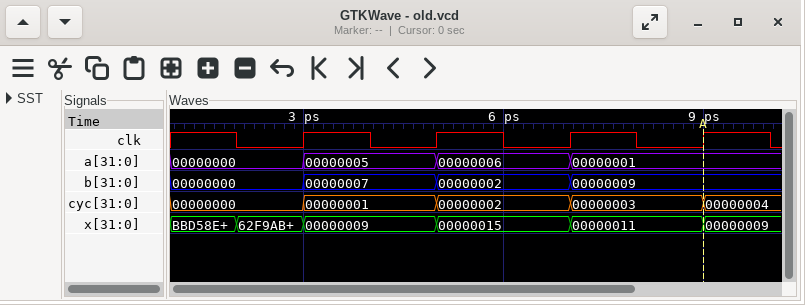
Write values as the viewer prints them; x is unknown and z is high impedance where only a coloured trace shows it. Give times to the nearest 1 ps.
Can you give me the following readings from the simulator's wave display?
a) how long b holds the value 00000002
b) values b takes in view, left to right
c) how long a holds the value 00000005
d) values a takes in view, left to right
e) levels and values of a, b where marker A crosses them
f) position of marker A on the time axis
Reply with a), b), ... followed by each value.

a) 2 ps
b) 00000000, 00000007, 00000002, 00000009
c) 2 ps
d) 00000000, 00000005, 00000006, 00000001
e) a=00000001, b=00000009
f) 9 ps
